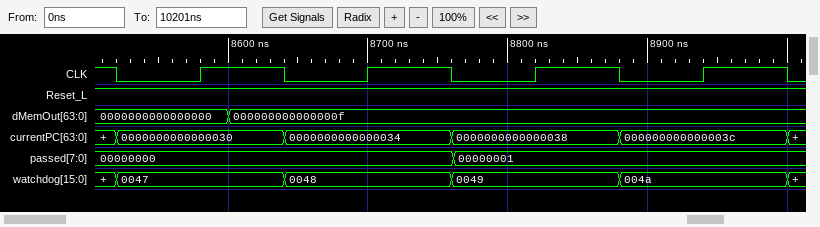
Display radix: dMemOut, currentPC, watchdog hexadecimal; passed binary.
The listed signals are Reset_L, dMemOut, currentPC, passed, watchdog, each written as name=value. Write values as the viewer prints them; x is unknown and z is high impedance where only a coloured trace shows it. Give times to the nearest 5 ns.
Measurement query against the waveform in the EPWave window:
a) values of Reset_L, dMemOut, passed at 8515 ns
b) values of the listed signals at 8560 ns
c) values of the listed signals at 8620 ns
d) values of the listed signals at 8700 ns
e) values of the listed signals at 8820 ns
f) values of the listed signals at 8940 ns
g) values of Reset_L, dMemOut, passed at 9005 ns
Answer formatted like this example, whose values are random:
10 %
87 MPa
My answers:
Reset_L=1, dMemOut=0000000000000000, passed=00000000
Reset_L=1, dMemOut=0000000000000000, currentPC=0000000000000030, passed=00000000, watchdog=0047
Reset_L=1, dMemOut=000000000000000f, currentPC=0000000000000030, passed=00000000, watchdog=0047
Reset_L=1, dMemOut=000000000000000f, currentPC=0000000000000034, passed=00000000, watchdog=0048
Reset_L=1, dMemOut=000000000000000f, currentPC=0000000000000038, passed=00000001, watchdog=0049
Reset_L=1, dMemOut=000000000000000f, currentPC=000000000000003c, passed=00000001, watchdog=004a
Reset_L=1, dMemOut=000000000000000f, passed=00000001
